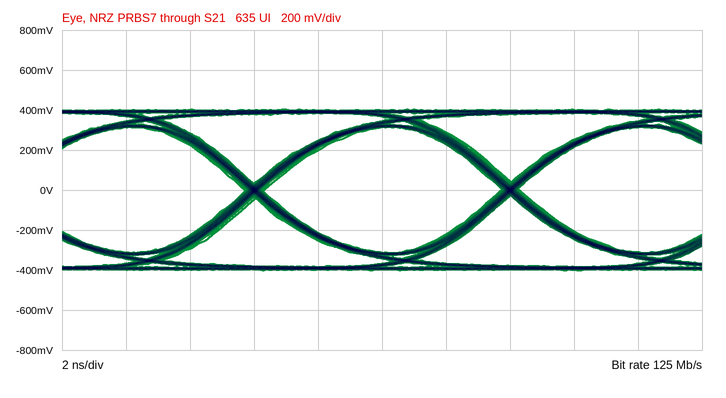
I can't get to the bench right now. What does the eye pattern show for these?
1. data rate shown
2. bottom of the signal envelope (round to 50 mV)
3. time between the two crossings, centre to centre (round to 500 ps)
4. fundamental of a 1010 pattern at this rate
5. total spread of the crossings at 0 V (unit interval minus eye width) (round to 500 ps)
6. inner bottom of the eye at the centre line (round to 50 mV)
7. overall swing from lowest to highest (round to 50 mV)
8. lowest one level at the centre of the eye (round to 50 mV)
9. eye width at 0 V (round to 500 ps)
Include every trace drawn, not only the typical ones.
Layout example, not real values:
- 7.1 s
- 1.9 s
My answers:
- 125 Mb/s
- -400 mV
- 8.0 ns
- 62.5 MHz
- 500 ps
- -300 mV
- 800 mV
- 300 mV
- 7.5 ns
